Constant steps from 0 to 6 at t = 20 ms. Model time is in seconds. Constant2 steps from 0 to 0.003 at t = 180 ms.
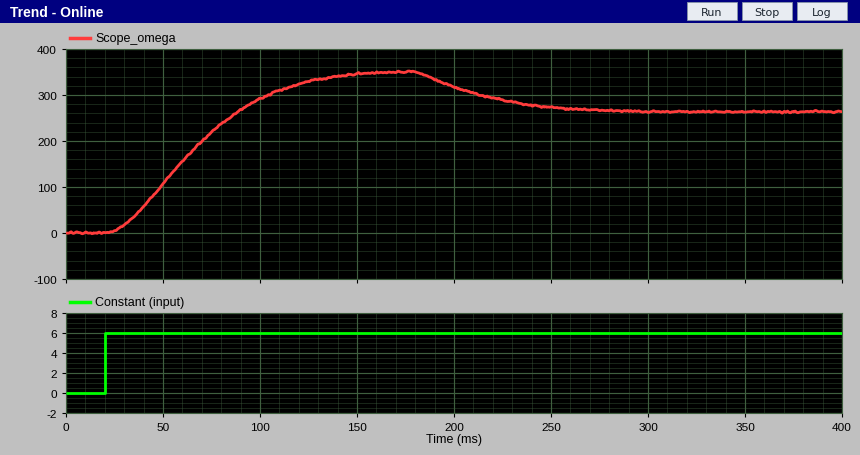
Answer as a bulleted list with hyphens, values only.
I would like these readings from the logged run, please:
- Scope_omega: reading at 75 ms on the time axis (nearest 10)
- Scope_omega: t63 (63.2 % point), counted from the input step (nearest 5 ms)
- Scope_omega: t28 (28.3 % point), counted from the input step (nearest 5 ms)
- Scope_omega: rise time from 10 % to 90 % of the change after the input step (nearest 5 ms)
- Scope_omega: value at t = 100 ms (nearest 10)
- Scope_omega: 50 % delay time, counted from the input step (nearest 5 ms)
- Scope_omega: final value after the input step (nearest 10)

- 220
- 55 ms
- 30 ms
- 80 ms
- 290
- 45 ms
- 350
